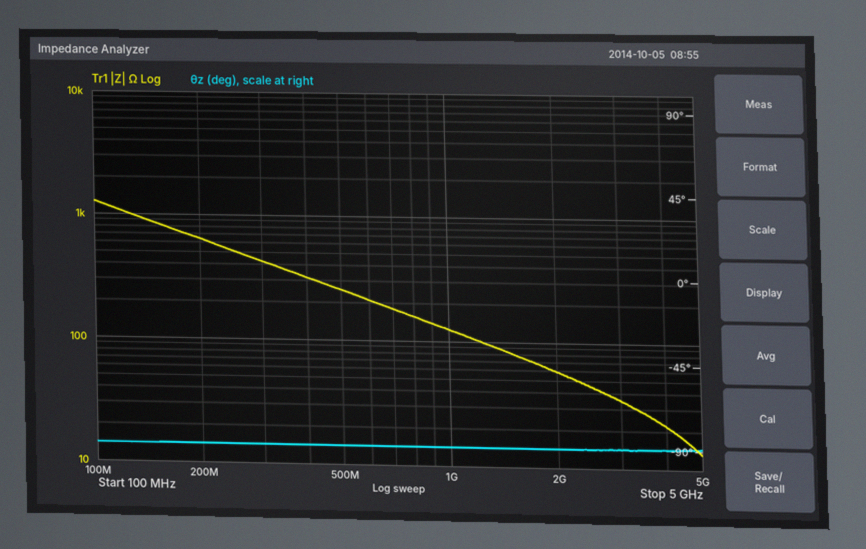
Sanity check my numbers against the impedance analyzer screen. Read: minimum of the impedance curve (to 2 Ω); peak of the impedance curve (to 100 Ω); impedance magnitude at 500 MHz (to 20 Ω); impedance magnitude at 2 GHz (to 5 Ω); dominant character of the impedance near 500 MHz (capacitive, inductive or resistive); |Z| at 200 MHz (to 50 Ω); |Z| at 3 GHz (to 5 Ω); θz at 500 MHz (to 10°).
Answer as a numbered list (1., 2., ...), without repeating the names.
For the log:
1. 14 Ω
2. 1.3 kΩ
3. 260 Ω
4. 60 Ω
5. capacitive
6. 650 Ω
7. 35 Ω
8. -90°
